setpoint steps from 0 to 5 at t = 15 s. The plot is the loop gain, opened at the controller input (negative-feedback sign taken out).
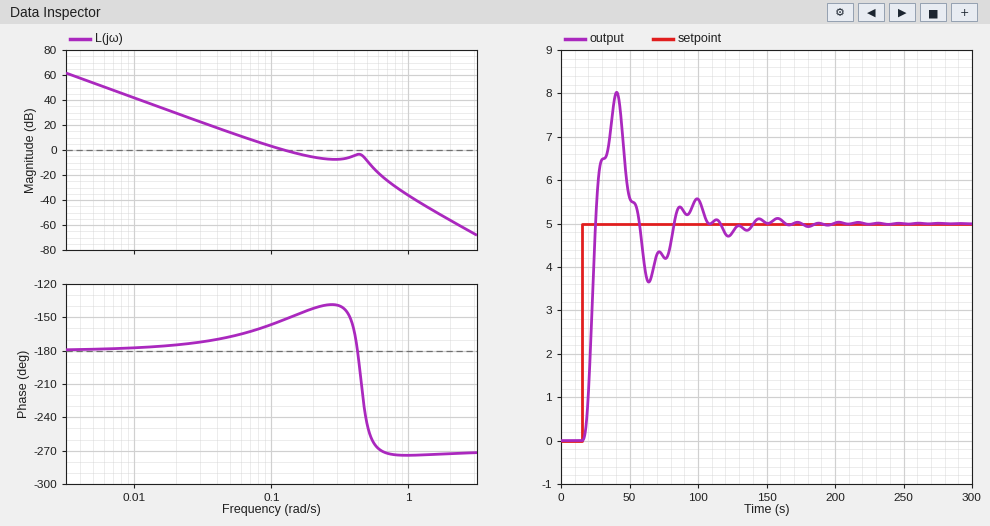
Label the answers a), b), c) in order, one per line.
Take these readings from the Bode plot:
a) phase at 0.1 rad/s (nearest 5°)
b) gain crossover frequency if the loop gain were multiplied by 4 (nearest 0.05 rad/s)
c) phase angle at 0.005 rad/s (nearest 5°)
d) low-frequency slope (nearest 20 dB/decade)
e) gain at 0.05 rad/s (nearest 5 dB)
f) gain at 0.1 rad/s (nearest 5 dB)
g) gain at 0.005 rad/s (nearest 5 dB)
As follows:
a) -155°
b) 0.55 rad/s
c) -180°
d) -40 dB/decade
e) 15 dB
f) 5 dB
g) 55 dB
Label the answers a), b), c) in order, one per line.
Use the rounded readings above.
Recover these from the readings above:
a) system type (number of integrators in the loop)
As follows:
a) 2
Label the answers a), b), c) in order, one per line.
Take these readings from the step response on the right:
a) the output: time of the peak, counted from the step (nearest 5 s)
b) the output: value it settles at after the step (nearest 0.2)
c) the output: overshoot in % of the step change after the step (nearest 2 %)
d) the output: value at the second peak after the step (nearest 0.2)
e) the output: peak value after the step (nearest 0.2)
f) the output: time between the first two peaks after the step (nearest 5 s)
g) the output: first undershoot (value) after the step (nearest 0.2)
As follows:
a) 25 s
b) 5.0
c) 60 %
d) 5.6
e) 8.0
f) 60 s
g) 3.6
